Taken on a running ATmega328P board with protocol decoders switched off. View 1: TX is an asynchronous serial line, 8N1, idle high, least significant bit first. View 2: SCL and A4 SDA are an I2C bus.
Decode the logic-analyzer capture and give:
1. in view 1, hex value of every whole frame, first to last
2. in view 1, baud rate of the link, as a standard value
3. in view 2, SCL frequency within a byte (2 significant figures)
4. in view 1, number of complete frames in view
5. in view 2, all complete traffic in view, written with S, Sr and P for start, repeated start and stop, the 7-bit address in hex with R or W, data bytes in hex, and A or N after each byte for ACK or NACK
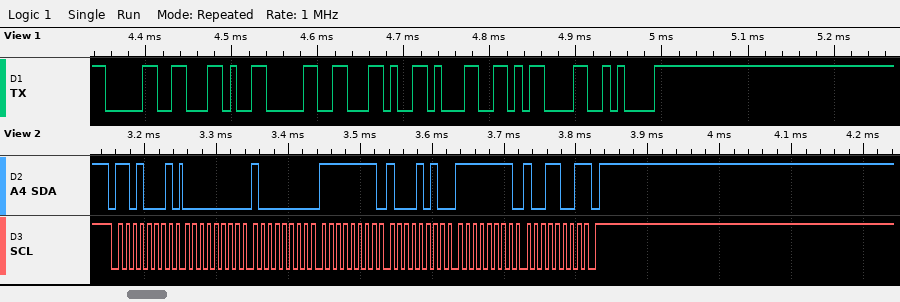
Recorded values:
30 2C 30 2C 31 0D 0A
115200 baud
100 kHz
7
S 68R A 00 A 80 A FF A 8A A FF A 99 N P
